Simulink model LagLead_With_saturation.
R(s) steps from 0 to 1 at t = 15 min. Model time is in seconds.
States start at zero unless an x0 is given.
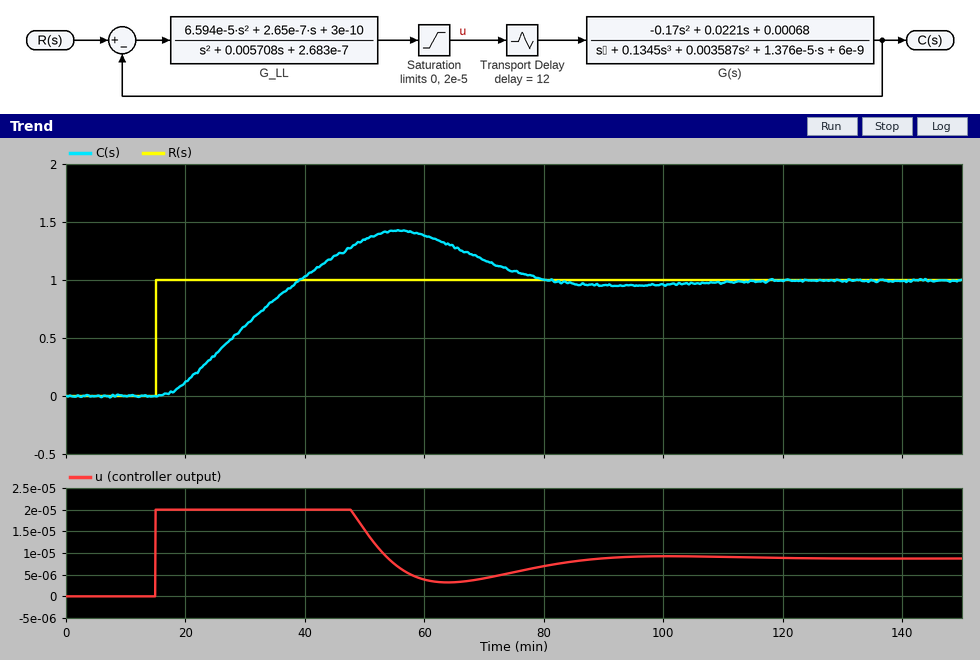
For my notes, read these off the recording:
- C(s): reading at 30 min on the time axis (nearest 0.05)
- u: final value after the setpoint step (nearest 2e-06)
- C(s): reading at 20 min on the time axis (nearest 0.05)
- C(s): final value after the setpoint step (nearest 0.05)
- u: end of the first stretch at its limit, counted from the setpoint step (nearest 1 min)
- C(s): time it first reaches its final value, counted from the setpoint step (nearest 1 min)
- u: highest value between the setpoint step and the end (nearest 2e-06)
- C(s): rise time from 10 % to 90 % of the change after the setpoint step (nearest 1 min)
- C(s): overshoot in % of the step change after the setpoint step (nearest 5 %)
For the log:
0.60
0.000008
0.10
1.00
33 min
24 min
0.000020
17 min
45 %
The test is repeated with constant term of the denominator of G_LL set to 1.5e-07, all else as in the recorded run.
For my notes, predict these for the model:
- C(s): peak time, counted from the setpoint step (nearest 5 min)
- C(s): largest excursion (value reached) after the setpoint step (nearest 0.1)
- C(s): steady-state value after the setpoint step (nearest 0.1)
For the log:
40 min
1.4
1.0
